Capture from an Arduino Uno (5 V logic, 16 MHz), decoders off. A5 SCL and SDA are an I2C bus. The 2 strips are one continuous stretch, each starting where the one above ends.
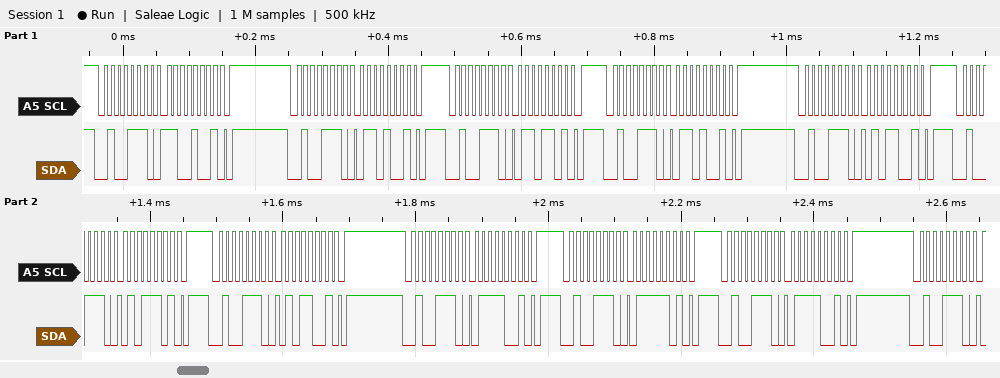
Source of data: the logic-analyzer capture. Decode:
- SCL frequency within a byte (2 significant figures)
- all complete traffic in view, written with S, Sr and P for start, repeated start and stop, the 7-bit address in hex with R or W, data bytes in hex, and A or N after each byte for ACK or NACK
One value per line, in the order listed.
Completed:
100 kHz
S 27W A C9 A P S 27W A 69 A P S 27W A 6D A P S 27W A 69 A P S 27W A 59 A P S 27W A 5D A P S 27W A 59 A P S 27W A 79 A P S 27W A 7D A P S 27W A 79 A P S 27W A
